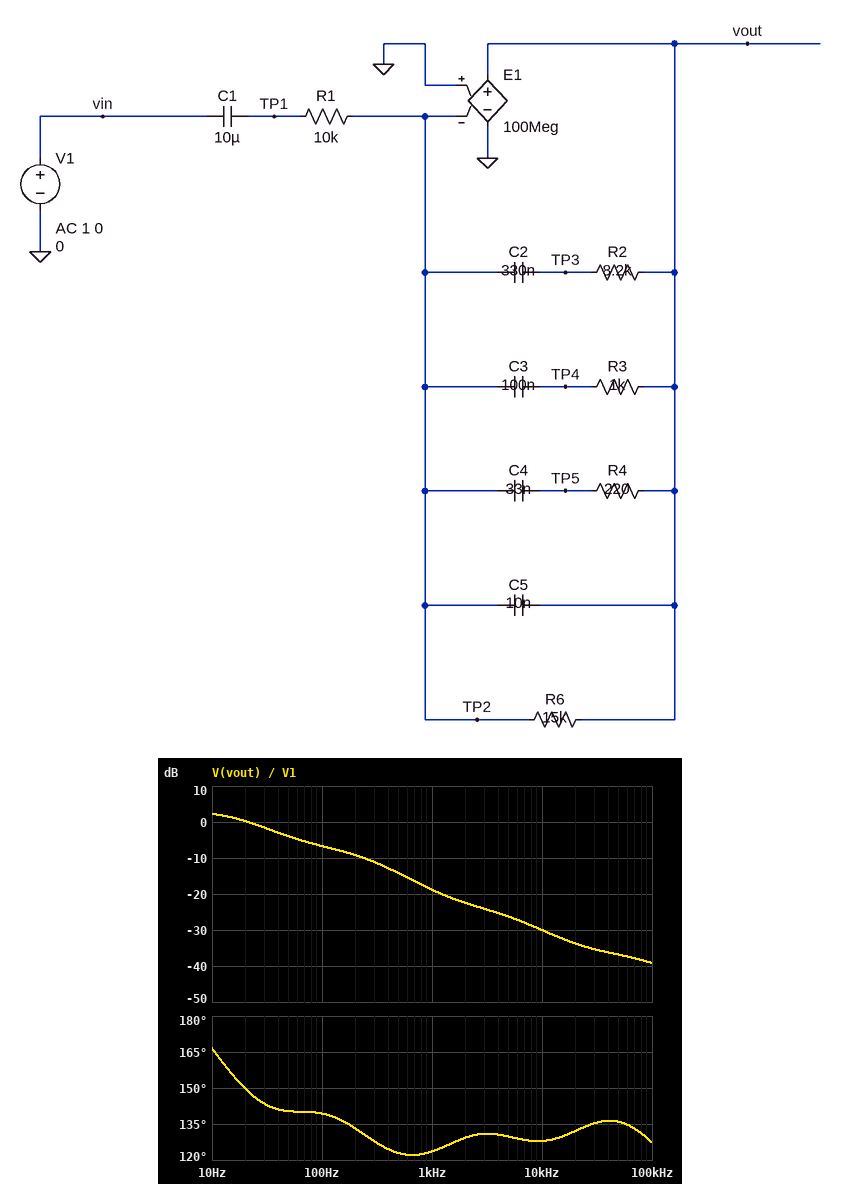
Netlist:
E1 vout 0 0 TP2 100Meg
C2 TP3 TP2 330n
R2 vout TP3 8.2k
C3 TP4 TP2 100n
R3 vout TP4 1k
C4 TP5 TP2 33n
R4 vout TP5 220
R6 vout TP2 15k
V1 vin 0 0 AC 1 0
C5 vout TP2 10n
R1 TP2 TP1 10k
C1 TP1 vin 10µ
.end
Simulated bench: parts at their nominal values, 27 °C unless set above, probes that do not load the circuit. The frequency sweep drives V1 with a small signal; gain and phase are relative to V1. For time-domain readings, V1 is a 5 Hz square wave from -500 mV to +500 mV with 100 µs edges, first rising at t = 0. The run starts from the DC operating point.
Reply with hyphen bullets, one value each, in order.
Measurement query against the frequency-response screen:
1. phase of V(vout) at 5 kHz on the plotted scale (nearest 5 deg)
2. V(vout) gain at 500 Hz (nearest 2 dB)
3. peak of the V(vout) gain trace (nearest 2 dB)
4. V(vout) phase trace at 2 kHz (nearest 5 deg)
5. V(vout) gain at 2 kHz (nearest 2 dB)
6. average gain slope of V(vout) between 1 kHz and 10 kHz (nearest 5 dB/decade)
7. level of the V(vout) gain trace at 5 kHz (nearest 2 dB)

- 130 deg
- -14 dB
- 2 dB
- 130 deg
- -22 dB
- -10 dB/decade
- -26 dB
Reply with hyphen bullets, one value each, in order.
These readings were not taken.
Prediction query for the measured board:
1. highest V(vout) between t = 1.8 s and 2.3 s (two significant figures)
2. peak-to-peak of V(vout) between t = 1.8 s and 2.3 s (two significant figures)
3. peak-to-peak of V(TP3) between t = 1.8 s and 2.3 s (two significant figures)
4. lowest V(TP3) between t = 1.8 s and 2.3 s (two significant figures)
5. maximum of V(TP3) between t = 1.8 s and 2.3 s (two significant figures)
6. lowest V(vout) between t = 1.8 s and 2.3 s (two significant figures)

- 840 mV
- 1.7 V
- 1.7 V
- -830 mV
- 830 mV
- -840 mV
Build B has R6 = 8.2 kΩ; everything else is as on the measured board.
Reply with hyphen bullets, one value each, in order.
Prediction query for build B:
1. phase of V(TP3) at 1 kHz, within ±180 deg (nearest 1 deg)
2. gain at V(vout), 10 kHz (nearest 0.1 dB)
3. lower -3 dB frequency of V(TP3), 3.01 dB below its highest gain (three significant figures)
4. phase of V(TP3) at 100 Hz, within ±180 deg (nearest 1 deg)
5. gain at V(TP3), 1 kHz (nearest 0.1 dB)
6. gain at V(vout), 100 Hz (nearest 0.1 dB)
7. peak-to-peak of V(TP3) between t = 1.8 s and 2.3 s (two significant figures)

- 40 deg
- -30.1 dB
- 1.43 Hz
- 88 deg
- -43.7 dB
- -8.3 dB
- 980 mV
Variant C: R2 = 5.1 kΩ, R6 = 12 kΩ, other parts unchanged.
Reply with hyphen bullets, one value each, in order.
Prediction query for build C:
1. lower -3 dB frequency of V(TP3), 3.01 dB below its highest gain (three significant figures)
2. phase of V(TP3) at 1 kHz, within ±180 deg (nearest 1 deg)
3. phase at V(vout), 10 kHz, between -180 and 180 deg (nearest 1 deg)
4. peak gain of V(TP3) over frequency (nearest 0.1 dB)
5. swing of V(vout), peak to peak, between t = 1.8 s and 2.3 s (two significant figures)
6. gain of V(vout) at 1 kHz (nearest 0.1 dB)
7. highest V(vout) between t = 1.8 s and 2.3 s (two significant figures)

- 1.41 Hz
- 43 deg
- 129 deg
- 1.0 dB
- 1.4 V
- -19.4 dB
- 700 mV
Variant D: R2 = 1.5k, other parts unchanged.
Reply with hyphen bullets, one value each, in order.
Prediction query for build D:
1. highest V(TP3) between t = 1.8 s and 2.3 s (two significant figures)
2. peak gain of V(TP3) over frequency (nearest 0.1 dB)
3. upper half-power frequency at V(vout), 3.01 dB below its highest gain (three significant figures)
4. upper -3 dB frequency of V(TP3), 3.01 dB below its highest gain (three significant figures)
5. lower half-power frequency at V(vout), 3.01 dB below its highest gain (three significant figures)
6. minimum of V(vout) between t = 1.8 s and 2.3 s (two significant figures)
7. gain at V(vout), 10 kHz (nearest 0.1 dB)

- 870 mV
- 2.9 dB
- 24.4 Hz
- 24.3 Hz
- 1.40 Hz
- -870 mV
- -31.0 dB
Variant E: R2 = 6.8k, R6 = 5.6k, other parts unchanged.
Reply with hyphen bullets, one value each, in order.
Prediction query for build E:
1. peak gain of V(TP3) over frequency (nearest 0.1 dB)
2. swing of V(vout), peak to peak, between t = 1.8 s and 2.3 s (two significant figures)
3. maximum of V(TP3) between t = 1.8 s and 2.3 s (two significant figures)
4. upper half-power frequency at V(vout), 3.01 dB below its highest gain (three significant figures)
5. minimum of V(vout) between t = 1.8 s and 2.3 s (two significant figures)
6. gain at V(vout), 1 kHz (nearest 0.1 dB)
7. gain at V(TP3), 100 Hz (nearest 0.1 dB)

- -5.4 dB
- 700 mV
- 350 mV
- 53.9 Hz
- -350 mV
- -19.6 dB
- -14.9 dB
